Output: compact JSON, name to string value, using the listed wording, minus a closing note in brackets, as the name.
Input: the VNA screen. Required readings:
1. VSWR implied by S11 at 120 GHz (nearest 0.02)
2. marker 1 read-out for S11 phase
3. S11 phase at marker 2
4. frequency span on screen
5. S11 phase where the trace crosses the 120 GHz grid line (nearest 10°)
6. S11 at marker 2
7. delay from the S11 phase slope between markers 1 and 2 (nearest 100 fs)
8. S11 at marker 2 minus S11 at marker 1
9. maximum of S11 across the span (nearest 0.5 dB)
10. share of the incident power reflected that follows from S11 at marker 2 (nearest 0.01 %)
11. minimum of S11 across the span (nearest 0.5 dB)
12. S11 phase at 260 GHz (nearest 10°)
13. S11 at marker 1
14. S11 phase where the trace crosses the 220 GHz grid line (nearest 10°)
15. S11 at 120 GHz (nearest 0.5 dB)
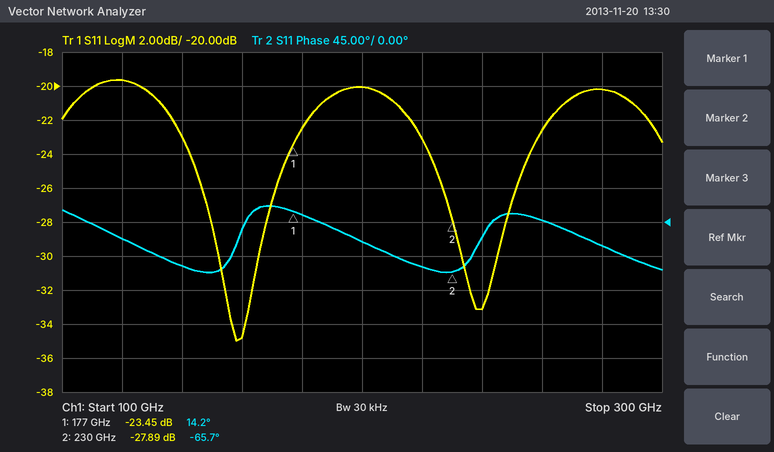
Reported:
{"VSWR implied by S11 at 120 GHz": "1.24", "marker 1 read-out for S11 phase": "14.2°", "S11 phase at marker 2": "-65.7°", "frequency span on screen": "200 GHz", "S11 phase where the trace crosses the 120 GHz grid line": "-20°", "S11 at marker 2": "-27.89 dB", "delay from the S11 phase slope between markers 1 and 2": "4.2 ps", "S11 at marker 2 minus S11 at marker 1": "-4.44 dB", "maximum of S11 across the span": "-19.5 dB", "share of the incident power reflected that follows from S11 at marker 2": "0.16 %", "minimum of S11 across the span": "-35.0 dB", "S11 phase at 260 GHz": "0°", "S11 at marker 1": "-23.45 dB", "S11 phase where the trace crosses the 220 GHz grid line": "-60°", "S11 at 120 GHz": "-19.5 dB"}
